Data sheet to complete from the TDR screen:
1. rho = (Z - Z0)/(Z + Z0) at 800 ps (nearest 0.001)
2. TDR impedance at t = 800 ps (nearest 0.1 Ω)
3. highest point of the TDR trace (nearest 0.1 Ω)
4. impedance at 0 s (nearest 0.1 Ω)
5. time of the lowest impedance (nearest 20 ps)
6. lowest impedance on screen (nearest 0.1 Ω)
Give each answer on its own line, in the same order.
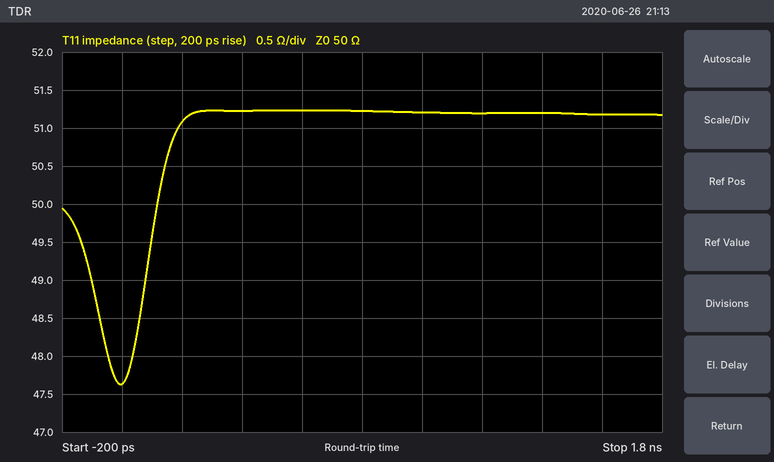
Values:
+0.012
51.2 Ω
51.2 Ω
47.6 Ω
0 ps
47.6 Ω
